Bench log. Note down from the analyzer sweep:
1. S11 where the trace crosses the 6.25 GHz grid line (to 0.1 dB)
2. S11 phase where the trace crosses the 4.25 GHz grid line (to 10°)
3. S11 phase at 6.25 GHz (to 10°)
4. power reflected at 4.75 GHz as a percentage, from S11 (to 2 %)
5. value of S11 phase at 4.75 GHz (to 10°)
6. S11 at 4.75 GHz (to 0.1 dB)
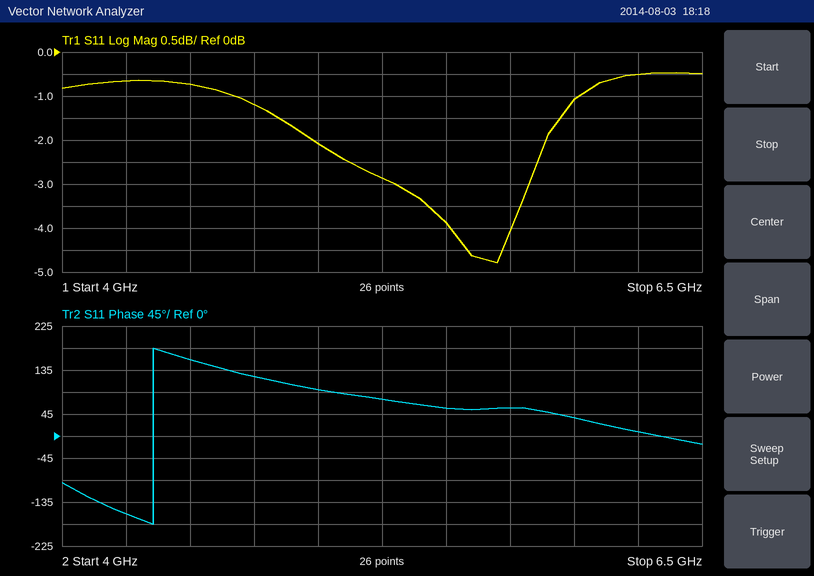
-0.5 dB
-160°
10°
76 %
120°
-1.2 dB
